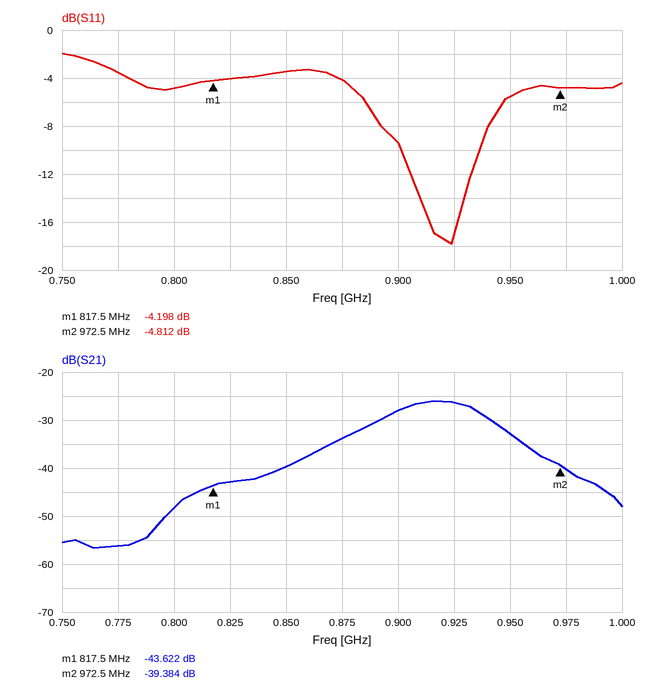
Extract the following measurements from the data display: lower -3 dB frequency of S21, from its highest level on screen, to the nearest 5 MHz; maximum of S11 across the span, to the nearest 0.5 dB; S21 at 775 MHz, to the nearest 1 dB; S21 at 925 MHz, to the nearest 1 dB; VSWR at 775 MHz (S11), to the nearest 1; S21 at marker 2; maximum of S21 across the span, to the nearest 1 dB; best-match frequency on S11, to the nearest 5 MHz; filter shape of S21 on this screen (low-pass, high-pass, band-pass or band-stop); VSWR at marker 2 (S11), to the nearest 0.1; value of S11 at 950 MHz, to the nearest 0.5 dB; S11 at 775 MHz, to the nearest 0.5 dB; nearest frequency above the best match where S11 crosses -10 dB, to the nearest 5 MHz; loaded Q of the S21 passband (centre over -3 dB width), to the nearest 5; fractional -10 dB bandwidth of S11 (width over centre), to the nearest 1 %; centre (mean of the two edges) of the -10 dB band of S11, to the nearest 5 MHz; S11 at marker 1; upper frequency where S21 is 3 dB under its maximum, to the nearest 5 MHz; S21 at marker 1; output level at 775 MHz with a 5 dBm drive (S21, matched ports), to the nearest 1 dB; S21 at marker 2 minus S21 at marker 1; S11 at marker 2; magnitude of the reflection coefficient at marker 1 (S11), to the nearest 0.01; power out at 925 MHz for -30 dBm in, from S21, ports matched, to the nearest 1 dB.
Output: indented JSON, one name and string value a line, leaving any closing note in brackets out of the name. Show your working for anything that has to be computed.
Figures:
{
  "lower -3 dB frequency of S21, from its highest level on screen, to the nearest 5 MHz": "895 MHz",
  "maximum of S11 across the span, to the nearest 0.5 dB": "-2.0 dB",
  "S21 at 775 MHz, to the nearest 1 dB": "-56 dB",
  "S21 at 925 MHz, to the nearest 1 dB": "-26 dB",
  "VSWR at 775 MHz (S11), to the nearest 1": "|Γ| = 10^(-3.5/20) = 0.6683; VSWR = (1 + 0.6683)/(1 − 0.6683) ≈ 5",
  "S21 at marker 2": "-39.384 dB",
  "maximum of S21 across the span, to the nearest 1 dB": "-26 dB",
  "best-match frequency on S11, to the nearest 5 MHz": "925 MHz",
  "filter shape of S21 on this screen": "band-pass",
  "VSWR at marker 2 (S11), to the nearest 0.1": "(1 + 0.5746)/(1 − 0.5746) ≈ 3.7",
  "value of S11 at 950 MHz, to the nearest 0.5 dB": "-5.5 dB",
  "S11 at 775 MHz, to the nearest 0.5 dB": "-3.5 dB",
  "nearest frequency above the best match where S11 crosses -10 dB, to the nearest 5 MHz": "935 MHz",
  "loaded Q of the S21 passband (centre over -3 dB width), to the nearest 5": "917.5 MHz / 45 MHz ≈ 20",
  "fractional -10 dB bandwidth of S11 (width over centre), to the nearest 1 %": "35 MHz / 917.5 MHz ≈ 4 %",
  "centre (mean of the two edges) of the -10 dB band of S11, to the nearest 5 MHz": "920 MHz",
  "S11 at marker 1": "-4.198 dB",
  "upper frequency where S21 is 3 dB under its maximum, to the nearest 5 MHz": "940 MHz",
  "S21 at marker 1": "-43.622 dB",
  "output level at 775 MHz with a 5 dBm drive (S21, matched ports), to the nearest 1 dB": "5 dBm + (-56 dB) = -51 dBm",
  "S21 at marker 2 minus S21 at marker 1": "-39.384 − (-43.622) = 4.238 dB",
  "S11 at marker 2": "-4.812 dB",
  "magnitude of the reflection coefficient at marker 1 (S11), to the nearest 0.01": "10^(-4.198/20) ≈ 0.62",
  "power out at 925 MHz for -30 dBm in, from S21, ports matched, to the nearest 1 dB": "-30 dBm + (-26 dB) = -56 dBm"
}
